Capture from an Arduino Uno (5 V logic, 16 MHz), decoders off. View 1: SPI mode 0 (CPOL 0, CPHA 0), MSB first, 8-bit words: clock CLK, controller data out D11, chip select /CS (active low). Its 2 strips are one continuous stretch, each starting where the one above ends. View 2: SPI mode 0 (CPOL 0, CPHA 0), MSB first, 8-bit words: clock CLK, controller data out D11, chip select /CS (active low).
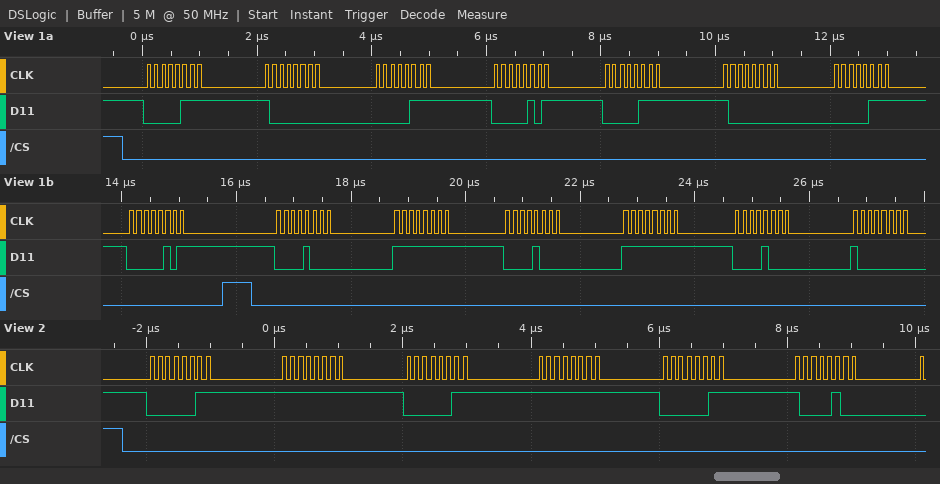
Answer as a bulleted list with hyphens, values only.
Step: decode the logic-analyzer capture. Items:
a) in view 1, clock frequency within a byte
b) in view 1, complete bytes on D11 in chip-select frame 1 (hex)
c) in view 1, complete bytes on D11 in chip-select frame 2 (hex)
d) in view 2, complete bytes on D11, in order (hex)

- 8 MHz
- 0x07 0x80 0x07 0x05 0x07 0x80 0x07 0x05
- 0x08 0xFF 0x08 0xFF 0x08 0x80
- 03 FF 03 FF 03 84
